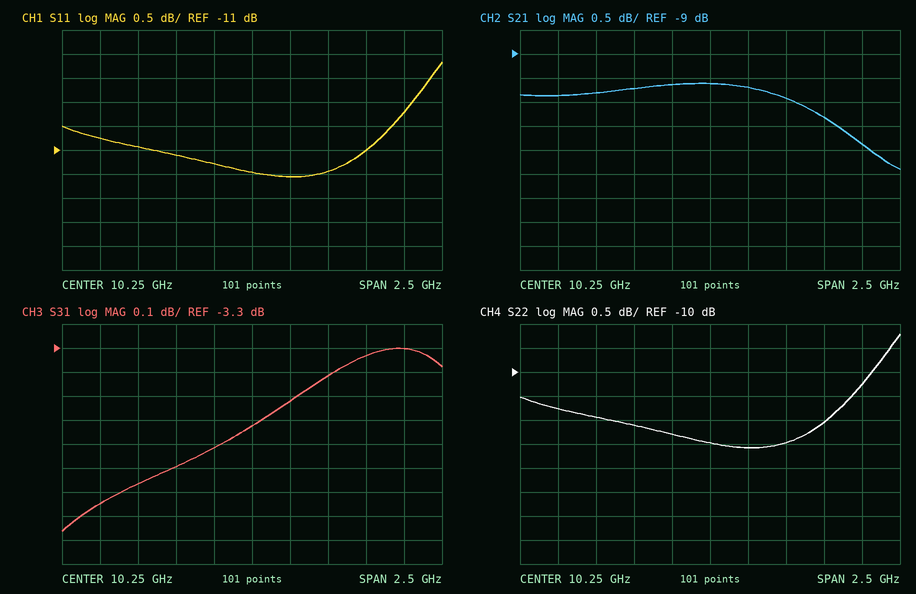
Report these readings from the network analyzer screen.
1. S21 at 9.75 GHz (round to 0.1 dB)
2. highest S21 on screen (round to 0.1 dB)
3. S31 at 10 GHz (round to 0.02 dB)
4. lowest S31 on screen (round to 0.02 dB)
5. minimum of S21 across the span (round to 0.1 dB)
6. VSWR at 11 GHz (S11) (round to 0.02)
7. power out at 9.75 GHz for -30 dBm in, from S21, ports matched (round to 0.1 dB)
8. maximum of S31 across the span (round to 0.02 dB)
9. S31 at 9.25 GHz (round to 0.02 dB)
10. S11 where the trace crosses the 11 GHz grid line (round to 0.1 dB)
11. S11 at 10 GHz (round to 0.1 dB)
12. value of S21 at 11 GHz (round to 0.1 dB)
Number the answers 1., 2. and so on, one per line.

1. -9.7 dB
2. -9.6 dB
3. -3.72 dB
4. -4.06 dB
5. -11.4 dB
6. 1.78
7. -39.7 dBm
8. -3.30 dB
9. -3.94 dB
10. -11.0 dB
11. -11.3 dB
12. -10.3 dB
